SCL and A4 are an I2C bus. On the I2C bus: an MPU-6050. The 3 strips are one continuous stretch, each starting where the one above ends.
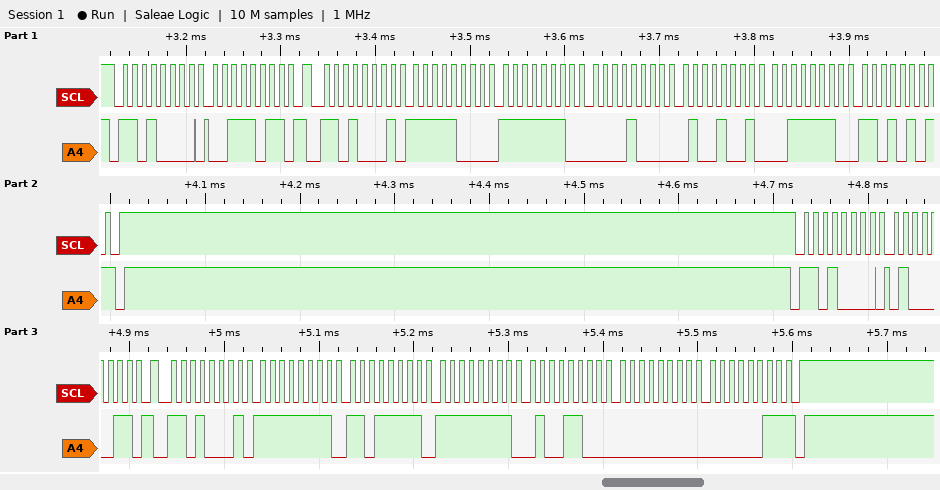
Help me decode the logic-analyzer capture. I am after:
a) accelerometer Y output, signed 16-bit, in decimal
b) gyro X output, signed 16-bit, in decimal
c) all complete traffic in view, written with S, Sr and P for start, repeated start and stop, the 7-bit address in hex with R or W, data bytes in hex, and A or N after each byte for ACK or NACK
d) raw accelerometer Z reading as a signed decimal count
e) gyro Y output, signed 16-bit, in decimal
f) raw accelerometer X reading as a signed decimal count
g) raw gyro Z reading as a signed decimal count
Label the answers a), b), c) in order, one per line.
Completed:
a) 2121
b) -33
c) S 68W A 3B A Sr 68R A F8 A FE A 08 A 49 A 3E A D5 N P S 68W A 43 A Sr 68R A FF A DF A FF A 4C A 00 A 03 N P
d) 16085
e) -180
f) -1794
g) 3
